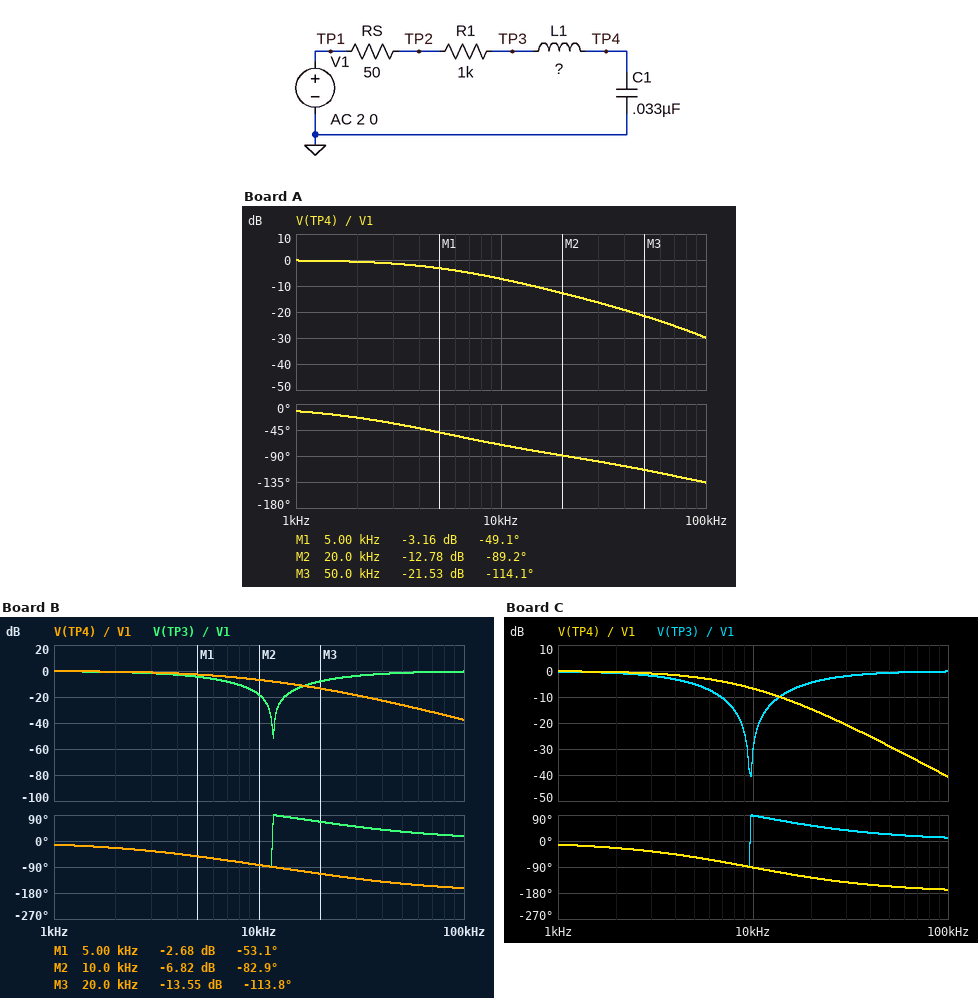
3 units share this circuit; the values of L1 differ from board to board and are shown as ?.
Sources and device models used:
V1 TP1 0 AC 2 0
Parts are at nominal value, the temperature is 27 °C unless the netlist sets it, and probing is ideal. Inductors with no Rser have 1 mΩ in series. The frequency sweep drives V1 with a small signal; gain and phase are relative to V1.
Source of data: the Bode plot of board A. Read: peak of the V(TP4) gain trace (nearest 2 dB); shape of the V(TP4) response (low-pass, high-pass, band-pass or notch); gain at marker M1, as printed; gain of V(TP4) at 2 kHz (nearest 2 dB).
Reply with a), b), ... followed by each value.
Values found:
a) 0 dB
b) low-pass
c) -3.16 dB
d) 0 dB
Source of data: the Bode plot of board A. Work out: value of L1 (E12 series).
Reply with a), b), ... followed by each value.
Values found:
a) 1.8 mH
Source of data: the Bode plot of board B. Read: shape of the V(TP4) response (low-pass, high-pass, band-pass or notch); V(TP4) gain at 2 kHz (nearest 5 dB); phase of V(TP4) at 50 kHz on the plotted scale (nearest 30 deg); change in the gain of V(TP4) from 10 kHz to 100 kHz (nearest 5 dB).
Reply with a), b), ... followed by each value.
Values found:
a) low-pass
b) 0 dB
c) -150 deg
d) -30 dB
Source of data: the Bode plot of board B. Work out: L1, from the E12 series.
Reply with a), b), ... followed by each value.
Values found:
a) 5.6 mH
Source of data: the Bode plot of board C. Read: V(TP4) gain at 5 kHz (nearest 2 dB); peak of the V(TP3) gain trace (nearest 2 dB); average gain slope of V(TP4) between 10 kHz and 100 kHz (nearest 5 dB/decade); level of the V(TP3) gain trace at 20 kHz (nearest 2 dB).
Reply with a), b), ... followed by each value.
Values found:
a) -2 dB
b) 0 dB
c) -35 dB/decade
d) -4 dB
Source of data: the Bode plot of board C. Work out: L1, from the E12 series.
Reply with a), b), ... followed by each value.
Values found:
a) 8.2 mH
